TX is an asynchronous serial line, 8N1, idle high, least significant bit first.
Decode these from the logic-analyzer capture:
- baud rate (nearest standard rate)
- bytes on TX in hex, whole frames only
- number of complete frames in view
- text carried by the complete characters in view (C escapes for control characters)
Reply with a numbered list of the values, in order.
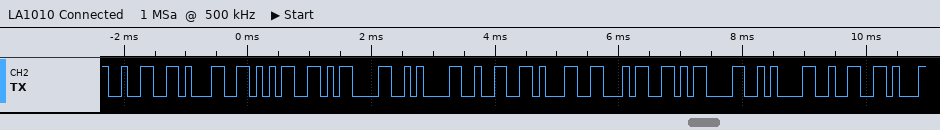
1. 9600 baud
2. 32 31 35 0D 0A 32 31 34 0D 0A 32
3. 11
4. "215\r\n214\r\n2"
